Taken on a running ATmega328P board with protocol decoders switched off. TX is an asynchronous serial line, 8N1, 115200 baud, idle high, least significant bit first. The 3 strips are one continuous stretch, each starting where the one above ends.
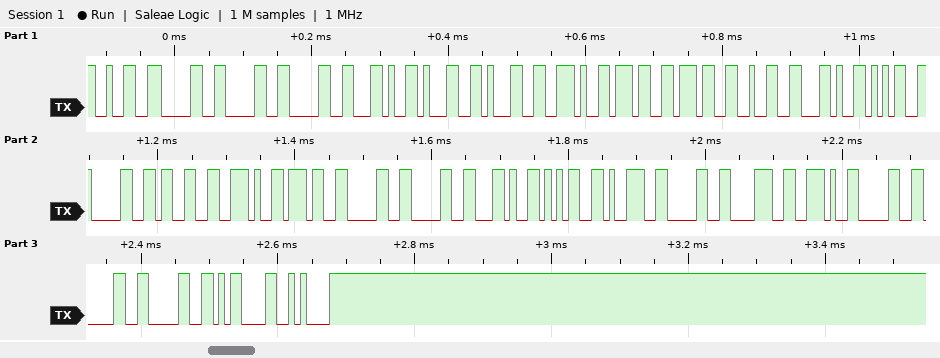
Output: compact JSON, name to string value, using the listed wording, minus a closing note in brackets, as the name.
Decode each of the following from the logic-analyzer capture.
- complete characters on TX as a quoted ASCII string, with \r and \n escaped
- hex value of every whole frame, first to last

{"complete characters on TX as a quoted ASCII string, with \\r and \\n escaped": "\"2000,11.772,503.700,5908.000\\r\\n\"", "hex value of every whole frame, first to last": "32 30 30 30 2C 31 31 2E 37 37 32 2C 35 30 33 2E 37 30 30 2C 35 39 30 38 2E 30 30 30 0D 0A"}
